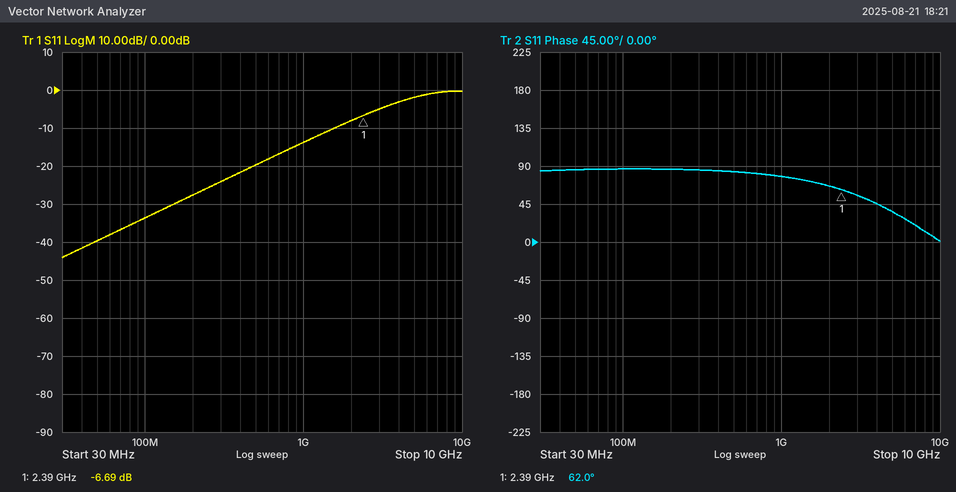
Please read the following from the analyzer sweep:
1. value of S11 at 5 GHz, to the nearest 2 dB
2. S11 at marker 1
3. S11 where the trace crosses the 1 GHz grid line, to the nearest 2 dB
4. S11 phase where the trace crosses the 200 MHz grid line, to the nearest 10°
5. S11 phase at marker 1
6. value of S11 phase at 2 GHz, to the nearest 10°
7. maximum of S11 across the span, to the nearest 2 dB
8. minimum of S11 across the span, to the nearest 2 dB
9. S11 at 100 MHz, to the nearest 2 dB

-2 dB
-6.69 dB
-14 dB
90°
62.0°
70°
0 dB
-44 dB
-34 dB
